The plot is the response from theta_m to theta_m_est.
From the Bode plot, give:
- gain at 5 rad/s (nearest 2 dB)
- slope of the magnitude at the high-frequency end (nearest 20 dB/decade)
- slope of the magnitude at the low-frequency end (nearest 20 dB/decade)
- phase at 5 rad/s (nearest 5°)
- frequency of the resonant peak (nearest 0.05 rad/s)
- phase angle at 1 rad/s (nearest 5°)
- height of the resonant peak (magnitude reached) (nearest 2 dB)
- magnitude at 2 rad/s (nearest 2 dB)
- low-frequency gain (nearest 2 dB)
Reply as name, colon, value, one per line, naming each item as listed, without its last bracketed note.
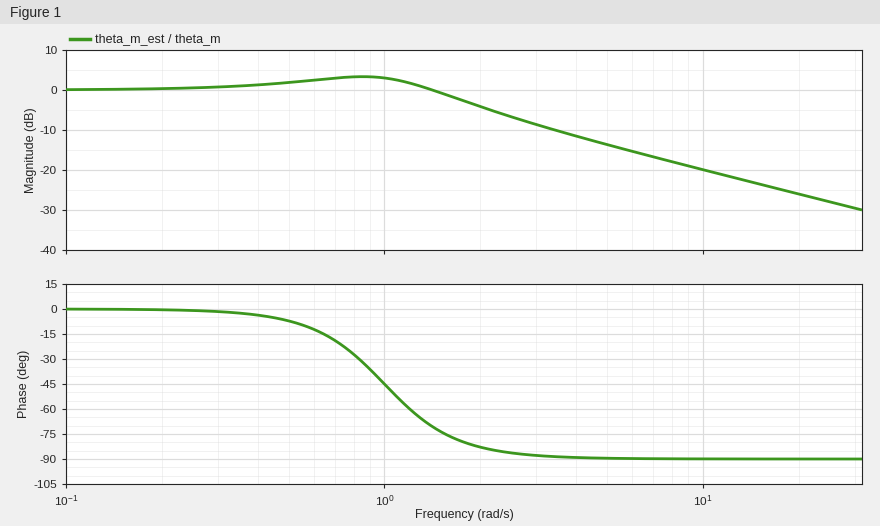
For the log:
gain at 5 rad/s: -14 dB
slope of the magnitude at the high-frequency end: -20 dB/decade
slope of the magnitude at the low-frequency end: 0 dB/decade
phase at 5 rad/s: -90°
frequency of the resonant peak: 0.85 rad/s
phase angle at 1 rad/s: -45°
height of the resonant peak (magnitude reached): 4 dB
magnitude at 2 rad/s: -4 dB
low-frequency gain: 0 dB
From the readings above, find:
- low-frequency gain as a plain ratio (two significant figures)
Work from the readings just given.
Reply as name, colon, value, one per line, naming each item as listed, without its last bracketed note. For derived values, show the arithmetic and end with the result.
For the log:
low-frequency gain as a plain ratio: 10^(0 / 20) = 1.0
